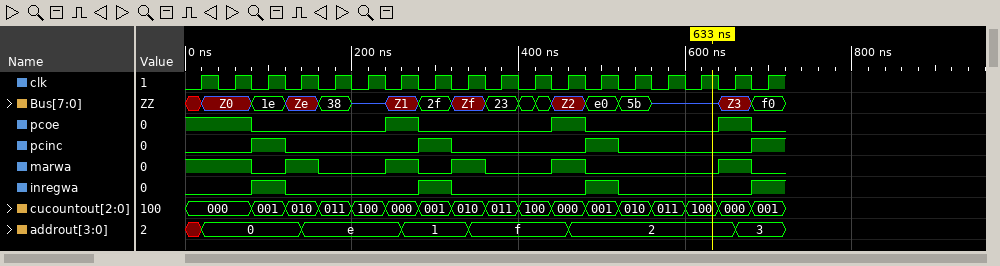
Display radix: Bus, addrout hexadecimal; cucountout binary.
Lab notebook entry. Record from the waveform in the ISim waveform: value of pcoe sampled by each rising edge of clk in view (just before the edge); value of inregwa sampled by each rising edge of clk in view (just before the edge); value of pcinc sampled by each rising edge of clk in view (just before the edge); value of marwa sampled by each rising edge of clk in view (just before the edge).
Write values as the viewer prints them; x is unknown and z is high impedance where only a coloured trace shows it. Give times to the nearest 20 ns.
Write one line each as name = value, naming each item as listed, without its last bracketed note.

value of pcoe sampled by each rising edge of clk in view = 1 1 0 0 0 0 1 0 0 0 0 1 0 0 0 0 1 0
value of inregwa sampled by each rising edge of clk in view = 0 0 1 0 0 0 0 1 0 0 0 0 1 0 0 0 0 1
value of pcinc sampled by each rising edge of clk in view = 0 0 1 0 0 0 0 1 0 0 0 0 1 0 0 0 0 1
value of marwa sampled by each rising edge of clk in view = 1 1 0 1 0 0 1 0 1 0 0 1 0 0 0 0 1 0
